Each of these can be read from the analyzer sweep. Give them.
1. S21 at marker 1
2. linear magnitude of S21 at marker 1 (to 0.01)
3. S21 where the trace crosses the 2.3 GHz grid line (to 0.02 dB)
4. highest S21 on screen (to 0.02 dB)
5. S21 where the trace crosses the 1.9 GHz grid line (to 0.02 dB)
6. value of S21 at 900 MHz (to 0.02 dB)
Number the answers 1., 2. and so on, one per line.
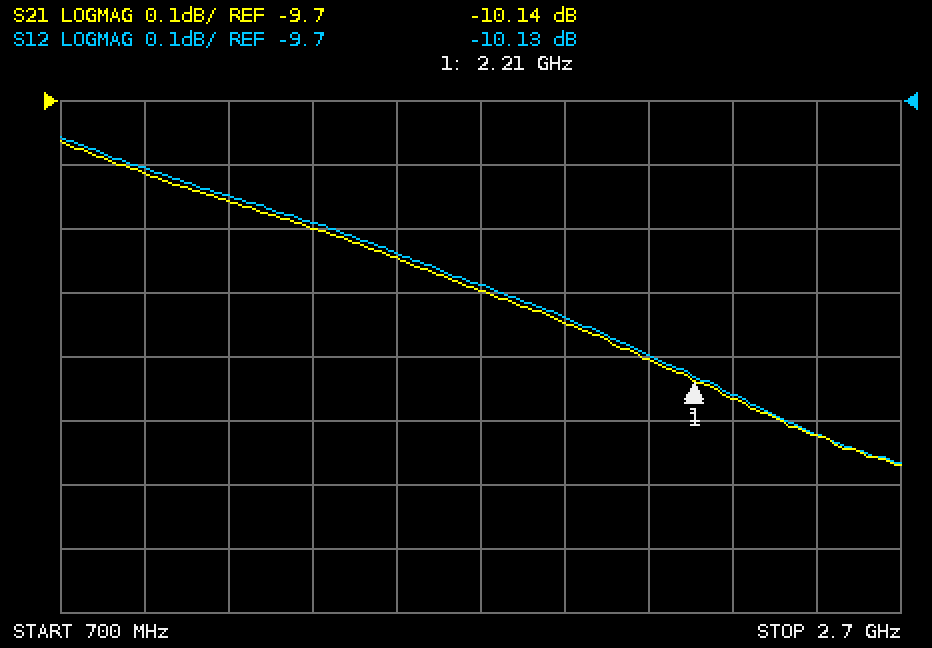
1. -10.14 dB
2. 0.31
3. -10.16 dB
4. -9.76 dB
5. -10.04 dB
6. -9.82 dB
